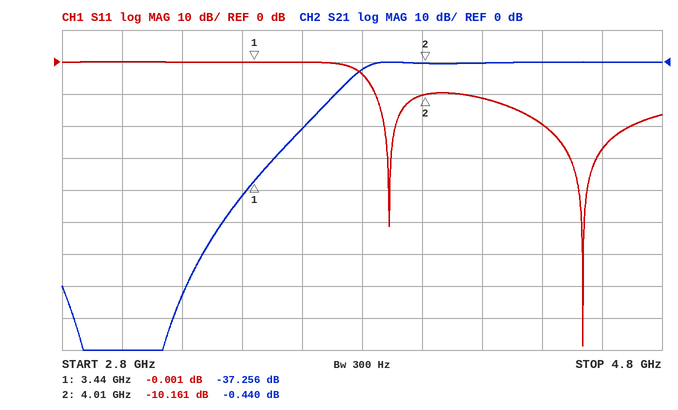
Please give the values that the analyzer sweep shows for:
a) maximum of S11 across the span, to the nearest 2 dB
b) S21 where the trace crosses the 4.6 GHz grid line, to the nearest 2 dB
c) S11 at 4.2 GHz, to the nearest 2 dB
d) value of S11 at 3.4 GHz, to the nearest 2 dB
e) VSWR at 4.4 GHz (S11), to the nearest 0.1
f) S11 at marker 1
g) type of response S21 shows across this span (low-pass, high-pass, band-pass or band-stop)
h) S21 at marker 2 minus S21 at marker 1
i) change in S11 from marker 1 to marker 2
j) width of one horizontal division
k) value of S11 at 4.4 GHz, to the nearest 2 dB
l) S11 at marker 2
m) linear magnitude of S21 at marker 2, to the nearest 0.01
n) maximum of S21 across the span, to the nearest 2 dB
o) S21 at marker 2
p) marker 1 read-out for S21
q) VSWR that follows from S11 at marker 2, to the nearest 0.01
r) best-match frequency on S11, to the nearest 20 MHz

0 dB
0 dB
-12 dB
0 dB
1.2
-0.001 dB
high-pass
36.816 dB
-10.160 dB
200 MHz
-20 dB
-10.161 dB
0.95
0 dB
-0.440 dB
-37.256 dB
1.90
4.54 GHz
